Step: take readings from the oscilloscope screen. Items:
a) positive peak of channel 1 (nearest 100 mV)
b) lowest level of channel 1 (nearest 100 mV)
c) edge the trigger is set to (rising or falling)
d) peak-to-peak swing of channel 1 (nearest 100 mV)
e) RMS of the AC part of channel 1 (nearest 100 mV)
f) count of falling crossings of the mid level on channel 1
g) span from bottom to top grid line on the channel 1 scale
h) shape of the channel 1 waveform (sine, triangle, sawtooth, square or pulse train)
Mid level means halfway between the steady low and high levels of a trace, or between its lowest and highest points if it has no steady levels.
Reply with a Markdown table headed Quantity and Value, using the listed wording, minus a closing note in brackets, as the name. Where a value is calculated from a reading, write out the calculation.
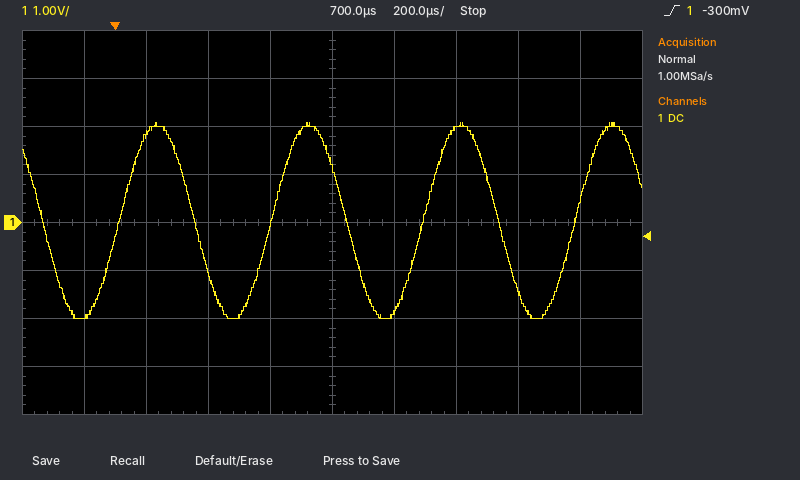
| Quantity | Value |
|---|---|
| positive peak of channel 1 | 2.1 V |
| lowest level of channel 1 | -2.0 V |
| edge the trigger is set to | rising |
| peak-to-peak swing of channel 1 | 2.1 V − (-2.0 V) = 4.1 V |
| RMS of the AC part of channel 1 | 4.1 V / (2√2) ≈ 1.4 V |
| count of falling crossings of the mid level on channel 1 | 4 |
| span from bottom to top grid line on the channel 1 scale | 8 V |
| shape of the channel 1 waveform | sine |
